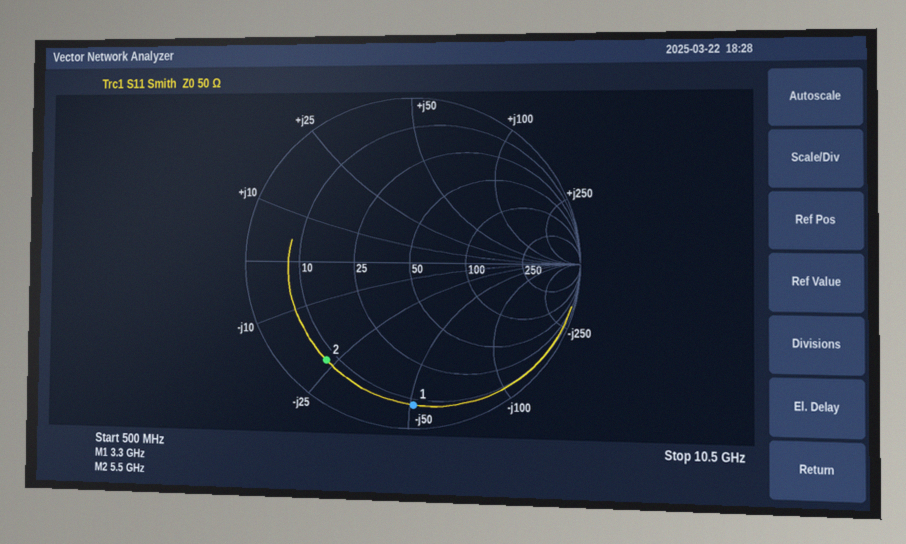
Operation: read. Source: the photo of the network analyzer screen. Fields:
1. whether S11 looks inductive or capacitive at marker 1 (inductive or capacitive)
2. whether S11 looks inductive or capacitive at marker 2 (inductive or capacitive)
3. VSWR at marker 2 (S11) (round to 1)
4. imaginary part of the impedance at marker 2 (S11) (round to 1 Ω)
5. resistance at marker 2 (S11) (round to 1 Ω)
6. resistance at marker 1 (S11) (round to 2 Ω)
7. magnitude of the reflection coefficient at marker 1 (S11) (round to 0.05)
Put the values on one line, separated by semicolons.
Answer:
capacitive; capacitive; 8; -23 Ω; 8 Ω; 8 Ω; 0.85
